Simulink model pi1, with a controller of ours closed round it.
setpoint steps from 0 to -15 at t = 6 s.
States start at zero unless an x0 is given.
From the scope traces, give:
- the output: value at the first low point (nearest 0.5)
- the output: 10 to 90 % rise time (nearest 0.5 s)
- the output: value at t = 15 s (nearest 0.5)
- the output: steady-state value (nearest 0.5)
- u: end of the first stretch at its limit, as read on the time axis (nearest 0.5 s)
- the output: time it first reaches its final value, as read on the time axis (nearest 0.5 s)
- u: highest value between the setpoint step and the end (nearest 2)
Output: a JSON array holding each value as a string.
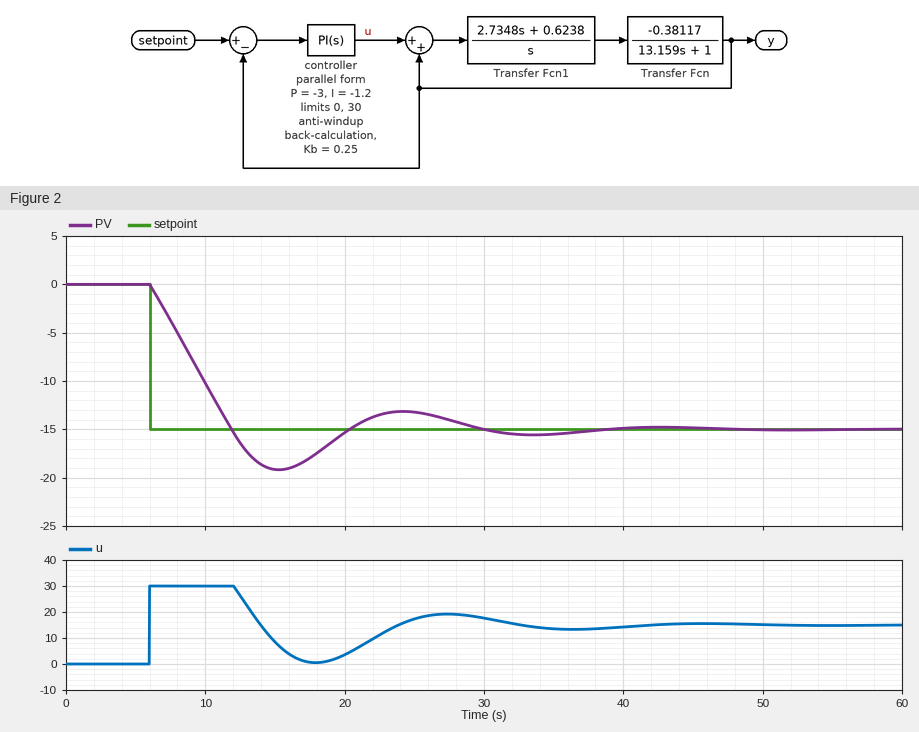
["-19.0", "4.5 s", "-19.0", "-15.0", "12.0 s", "12.0 s", "30"]
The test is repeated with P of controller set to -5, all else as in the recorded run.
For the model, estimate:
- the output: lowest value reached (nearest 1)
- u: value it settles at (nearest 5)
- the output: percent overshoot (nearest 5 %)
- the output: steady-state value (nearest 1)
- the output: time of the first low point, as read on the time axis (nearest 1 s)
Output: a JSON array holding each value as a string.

["-17", "15", "15 %", "-15", "15 s"]
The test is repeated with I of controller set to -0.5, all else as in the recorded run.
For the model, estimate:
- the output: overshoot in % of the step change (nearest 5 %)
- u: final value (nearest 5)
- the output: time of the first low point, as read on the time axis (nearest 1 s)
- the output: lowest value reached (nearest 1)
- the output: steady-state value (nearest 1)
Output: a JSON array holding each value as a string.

["10 %", "15", "16 s", "-17", "-15"]
